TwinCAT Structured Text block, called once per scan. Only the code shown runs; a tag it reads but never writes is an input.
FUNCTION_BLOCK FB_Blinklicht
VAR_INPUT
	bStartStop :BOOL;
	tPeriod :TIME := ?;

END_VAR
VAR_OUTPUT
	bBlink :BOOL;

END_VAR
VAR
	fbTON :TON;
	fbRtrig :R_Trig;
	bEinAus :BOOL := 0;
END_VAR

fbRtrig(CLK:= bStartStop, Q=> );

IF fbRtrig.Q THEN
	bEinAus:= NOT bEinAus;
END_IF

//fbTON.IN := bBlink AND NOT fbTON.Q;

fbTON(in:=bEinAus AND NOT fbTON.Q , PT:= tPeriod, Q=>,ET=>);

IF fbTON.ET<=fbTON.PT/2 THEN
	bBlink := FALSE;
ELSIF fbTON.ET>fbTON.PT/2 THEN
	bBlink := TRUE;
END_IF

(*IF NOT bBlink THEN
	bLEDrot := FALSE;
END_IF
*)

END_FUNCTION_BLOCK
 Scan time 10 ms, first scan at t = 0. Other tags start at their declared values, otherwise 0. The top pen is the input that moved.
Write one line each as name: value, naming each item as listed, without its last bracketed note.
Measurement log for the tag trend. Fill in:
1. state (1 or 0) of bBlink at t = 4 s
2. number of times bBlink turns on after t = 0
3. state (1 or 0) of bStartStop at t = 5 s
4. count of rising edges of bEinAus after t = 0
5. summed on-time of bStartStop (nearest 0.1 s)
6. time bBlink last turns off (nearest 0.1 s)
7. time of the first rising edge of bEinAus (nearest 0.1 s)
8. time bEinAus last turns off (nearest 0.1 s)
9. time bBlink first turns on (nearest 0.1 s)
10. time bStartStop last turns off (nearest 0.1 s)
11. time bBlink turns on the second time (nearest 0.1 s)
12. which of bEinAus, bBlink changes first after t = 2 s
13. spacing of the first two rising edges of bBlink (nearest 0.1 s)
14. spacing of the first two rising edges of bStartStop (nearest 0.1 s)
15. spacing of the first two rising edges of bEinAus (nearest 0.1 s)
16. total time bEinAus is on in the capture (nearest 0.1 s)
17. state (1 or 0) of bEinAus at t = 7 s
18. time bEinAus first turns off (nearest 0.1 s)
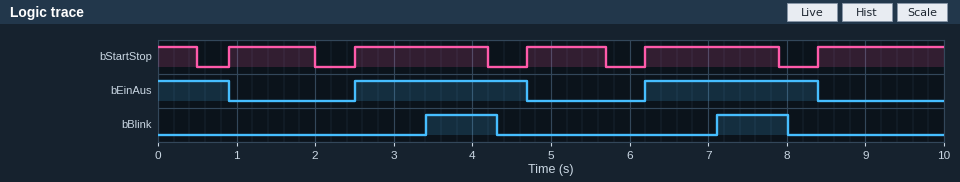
state (1 or 0) of bBlink at t = 4 s: 1
number of times bBlink turns on after t = 0: 2
state (1 or 0) of bStartStop at t = 5 s: 1
count of rising edges of bEinAus after t = 0: 2
summed on-time of bStartStop: 7.6 s
time bBlink last turns off: 8.0 s
time of the first rising edge of bEinAus: 2.5 s
time bEinAus last turns off: 8.4 s
time bBlink first turns on: 3.4 s
time bStartStop last turns off: 7.9 s
time bBlink turns on the second time: 7.1 s
which of bEinAus, bBlink changes first after t = 2 s: bEinAus
spacing of the first two rising edges of bBlink: 3.7 s
spacing of the first two rising edges of bStartStop: 1.6 s
spacing of the first two rising edges of bEinAus: 3.7 s
total time bEinAus is on in the capture: 5.3 s
state (1 or 0) of bEinAus at t = 7 s: 1
time bEinAus first turns off: 0.9 s
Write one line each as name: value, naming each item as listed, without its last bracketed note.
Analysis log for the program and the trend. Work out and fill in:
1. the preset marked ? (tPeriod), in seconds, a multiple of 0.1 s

the preset marked ? (tPeriod), in seconds, a multiple of 0.1 s: 1.8 s
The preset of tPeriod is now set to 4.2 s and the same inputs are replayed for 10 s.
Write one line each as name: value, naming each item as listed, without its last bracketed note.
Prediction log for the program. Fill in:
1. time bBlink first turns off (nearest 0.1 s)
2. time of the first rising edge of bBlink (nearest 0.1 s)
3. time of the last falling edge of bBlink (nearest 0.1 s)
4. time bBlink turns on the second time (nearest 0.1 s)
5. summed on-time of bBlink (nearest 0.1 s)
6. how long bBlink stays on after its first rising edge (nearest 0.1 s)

time bBlink first turns off: 4.7 s
time of the first rising edge of bBlink: 4.6 s
time of the last falling edge of bBlink: 8.4 s
time bBlink turns on the second time: 8.3 s
summed on-time of bBlink: 0.2 s
how long bBlink stays on after its first rising edge: 0.1 s
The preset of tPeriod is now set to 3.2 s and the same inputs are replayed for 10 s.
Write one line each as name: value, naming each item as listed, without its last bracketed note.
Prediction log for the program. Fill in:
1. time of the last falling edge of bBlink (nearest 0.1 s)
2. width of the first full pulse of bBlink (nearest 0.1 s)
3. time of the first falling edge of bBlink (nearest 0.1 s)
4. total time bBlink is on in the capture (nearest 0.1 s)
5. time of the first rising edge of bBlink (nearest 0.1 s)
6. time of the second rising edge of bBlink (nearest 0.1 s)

time of the last falling edge of bBlink: 8.4 s
width of the first full pulse of bBlink: 0.6 s
time of the first falling edge of bBlink: 4.7 s
total time bBlink is on in the capture: 1.2 s
time of the first rising edge of bBlink: 4.1 s
time of the second rising edge of bBlink: 7.8 s
